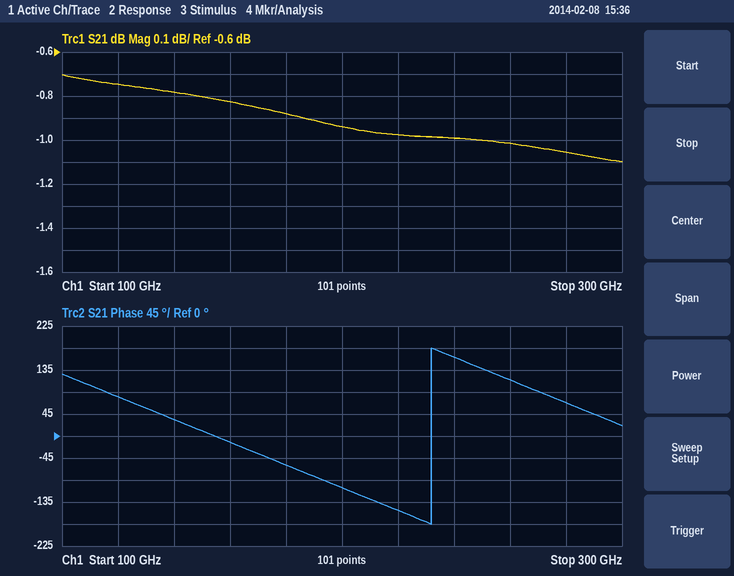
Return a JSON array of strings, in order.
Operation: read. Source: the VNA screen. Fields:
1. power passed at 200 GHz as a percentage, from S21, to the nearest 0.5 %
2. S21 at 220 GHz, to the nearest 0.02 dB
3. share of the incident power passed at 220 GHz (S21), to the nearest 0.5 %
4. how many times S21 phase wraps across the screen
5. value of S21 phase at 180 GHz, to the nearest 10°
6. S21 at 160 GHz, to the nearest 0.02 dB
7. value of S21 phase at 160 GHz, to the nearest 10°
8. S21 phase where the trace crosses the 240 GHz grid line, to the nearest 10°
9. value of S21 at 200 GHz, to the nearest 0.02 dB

["80.5 %", "-0.98 dB", "80.0 %", "1", "-60°", "-0.82 dB", "-10°", "160°", "-0.94 dB"]
